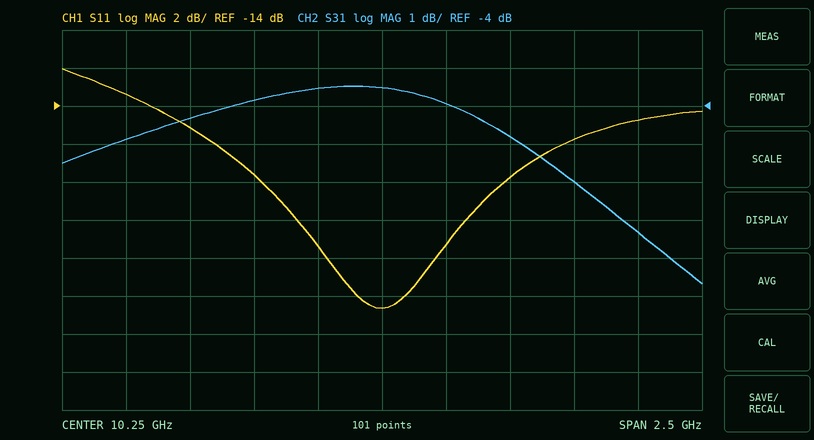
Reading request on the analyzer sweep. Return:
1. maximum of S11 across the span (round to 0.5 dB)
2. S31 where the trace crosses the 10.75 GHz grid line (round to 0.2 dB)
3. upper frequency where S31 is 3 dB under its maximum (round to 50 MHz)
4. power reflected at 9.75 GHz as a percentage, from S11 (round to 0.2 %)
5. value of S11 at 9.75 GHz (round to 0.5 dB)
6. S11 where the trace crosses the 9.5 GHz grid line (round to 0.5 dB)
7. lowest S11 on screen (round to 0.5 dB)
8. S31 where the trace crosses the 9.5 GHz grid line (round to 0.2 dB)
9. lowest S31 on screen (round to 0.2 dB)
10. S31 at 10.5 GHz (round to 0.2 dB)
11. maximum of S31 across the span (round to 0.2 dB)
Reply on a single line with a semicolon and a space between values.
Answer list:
-12.0 dB; -4.8 dB; 11.10 GHz; 1.8 %; -17.5 dB; -15.0 dB; -24.5 dB; -4.4 dB; -8.6 dB; -4.0 dB; -3.4 dB
